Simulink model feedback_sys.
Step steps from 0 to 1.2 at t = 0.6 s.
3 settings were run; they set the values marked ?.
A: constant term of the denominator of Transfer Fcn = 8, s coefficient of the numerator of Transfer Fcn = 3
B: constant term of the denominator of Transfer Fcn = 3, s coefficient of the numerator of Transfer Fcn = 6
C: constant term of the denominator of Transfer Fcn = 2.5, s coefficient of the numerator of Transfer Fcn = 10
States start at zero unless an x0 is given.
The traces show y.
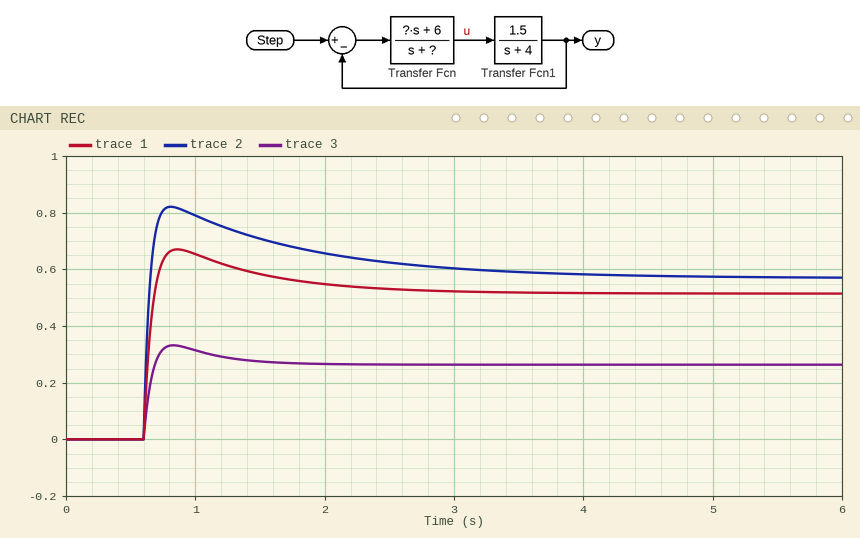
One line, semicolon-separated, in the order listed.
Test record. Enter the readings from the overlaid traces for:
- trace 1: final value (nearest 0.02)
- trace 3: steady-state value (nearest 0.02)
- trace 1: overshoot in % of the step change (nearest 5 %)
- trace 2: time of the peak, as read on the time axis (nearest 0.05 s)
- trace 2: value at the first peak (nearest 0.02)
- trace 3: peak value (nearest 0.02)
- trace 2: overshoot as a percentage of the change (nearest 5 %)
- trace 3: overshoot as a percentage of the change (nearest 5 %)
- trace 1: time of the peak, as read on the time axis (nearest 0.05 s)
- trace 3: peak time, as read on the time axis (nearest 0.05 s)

0.52; 0.26; 30 %; 0.80 s; 0.82; 0.34; 45 %; 25 %; 0.85 s; 0.85 s
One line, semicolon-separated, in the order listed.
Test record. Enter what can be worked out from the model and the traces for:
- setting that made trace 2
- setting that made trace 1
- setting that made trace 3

C; B; A
